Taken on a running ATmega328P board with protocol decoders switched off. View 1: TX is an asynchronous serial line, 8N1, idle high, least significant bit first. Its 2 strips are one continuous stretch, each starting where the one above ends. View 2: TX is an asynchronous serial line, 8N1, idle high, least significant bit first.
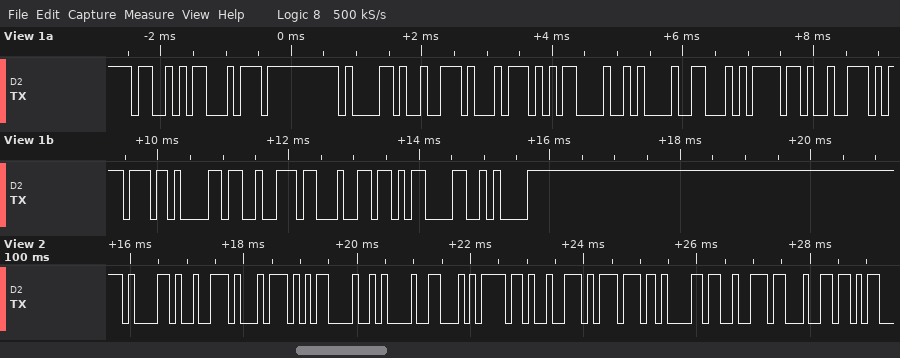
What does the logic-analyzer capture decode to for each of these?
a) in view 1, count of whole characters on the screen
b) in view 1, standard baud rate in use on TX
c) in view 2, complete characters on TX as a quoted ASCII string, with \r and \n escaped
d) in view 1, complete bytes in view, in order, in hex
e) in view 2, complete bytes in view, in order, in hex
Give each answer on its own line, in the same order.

16
9600 baud
"art\r\nForward"
53 74 61 72 74 0D 0A 46 6F 72 77 61 72 64 0D 0A
0x61 0x72 0x74 0x0D 0x0A 0x46 0x6F 0x72 0x77 0x61 0x72 0x64
